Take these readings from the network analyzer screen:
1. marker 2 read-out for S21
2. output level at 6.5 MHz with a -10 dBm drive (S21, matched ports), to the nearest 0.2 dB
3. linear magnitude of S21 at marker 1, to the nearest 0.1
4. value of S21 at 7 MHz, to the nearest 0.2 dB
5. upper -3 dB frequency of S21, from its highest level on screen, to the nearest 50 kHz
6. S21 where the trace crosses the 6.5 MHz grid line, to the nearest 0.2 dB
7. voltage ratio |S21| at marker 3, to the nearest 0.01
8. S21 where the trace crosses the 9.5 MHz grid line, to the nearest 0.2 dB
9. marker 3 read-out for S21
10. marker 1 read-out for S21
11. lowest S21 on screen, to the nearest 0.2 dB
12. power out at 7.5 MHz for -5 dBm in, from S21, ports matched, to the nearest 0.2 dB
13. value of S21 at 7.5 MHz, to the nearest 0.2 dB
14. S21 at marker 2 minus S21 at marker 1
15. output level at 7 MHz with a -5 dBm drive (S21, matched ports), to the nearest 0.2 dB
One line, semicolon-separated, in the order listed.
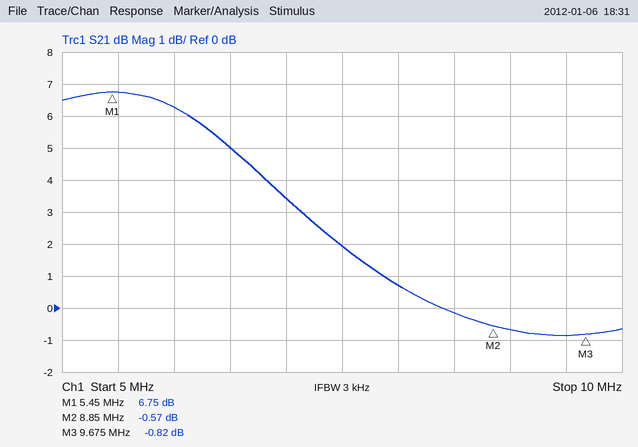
-0.57 dB; -5.0 dBm; 2.2; 3.4 dB; 6.90 MHz; 5.0 dB; 0.91; -0.8 dB; -0.82 dB; 6.75 dB; -0.8 dB; -3.0 dBm; 2.0 dB; -7.32 dB; -1.6 dBm
